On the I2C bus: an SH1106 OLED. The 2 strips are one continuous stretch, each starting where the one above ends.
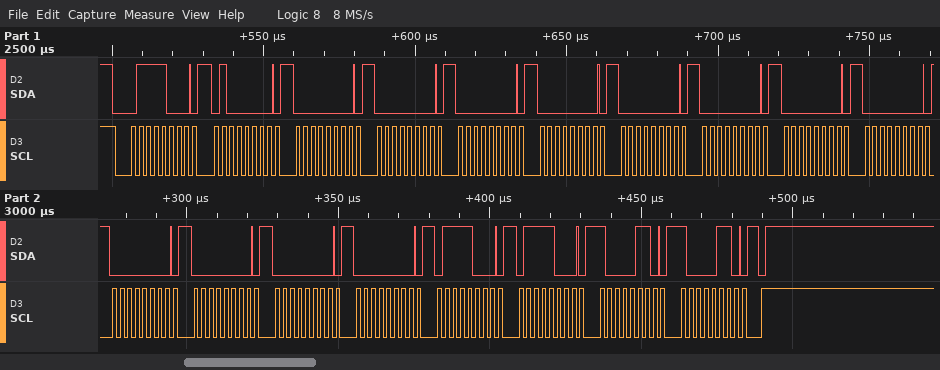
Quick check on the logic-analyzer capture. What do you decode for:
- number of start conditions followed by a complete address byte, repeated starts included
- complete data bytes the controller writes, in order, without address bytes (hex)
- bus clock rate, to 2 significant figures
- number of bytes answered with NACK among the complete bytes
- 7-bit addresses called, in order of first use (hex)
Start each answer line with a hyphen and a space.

- 1
- 40 00 00 00 00 00 00 00 00 00 00 00 00 78 78 86 86
- 400 kHz
- 0
- 0x3C
